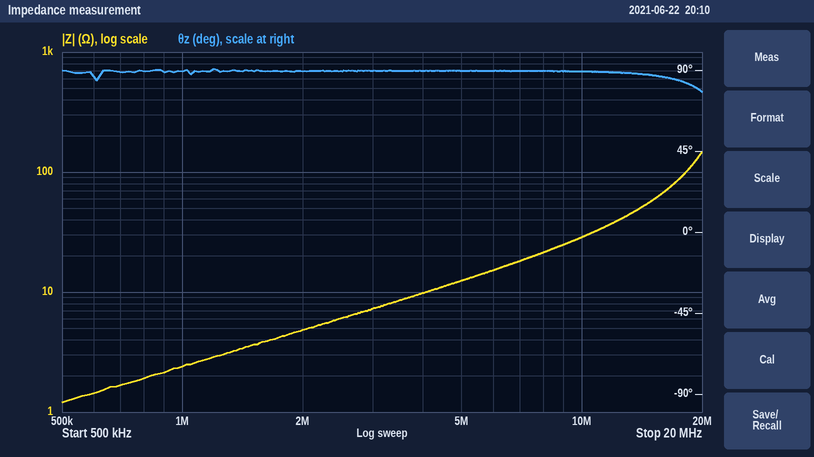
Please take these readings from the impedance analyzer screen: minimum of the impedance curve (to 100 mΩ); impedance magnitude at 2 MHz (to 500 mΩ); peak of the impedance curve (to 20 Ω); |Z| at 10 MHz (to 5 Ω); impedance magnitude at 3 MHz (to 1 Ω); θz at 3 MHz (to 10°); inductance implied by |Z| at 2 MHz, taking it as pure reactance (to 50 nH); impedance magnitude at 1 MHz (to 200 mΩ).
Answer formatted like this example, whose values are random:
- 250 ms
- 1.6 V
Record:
- 1.2 Ω
- 5.0 Ω
- 140 Ω
- 30 Ω
- 7 Ω
- 90°
- 400 nH
- 2.4 Ω
